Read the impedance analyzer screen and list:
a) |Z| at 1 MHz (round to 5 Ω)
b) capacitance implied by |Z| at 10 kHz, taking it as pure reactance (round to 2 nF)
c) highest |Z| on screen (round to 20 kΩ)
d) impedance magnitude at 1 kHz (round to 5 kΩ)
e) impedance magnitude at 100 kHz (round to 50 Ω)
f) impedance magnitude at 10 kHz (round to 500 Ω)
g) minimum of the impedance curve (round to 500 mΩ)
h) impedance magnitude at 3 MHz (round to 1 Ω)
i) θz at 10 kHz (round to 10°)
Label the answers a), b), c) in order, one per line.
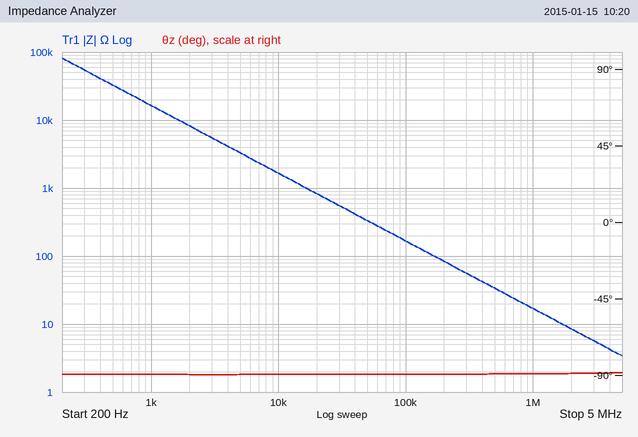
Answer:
a) 15 Ω
b) 10 nF
c) 80 kΩ
d) 15 kΩ
e) 150 Ω
f) 1.5 kΩ
g) 3.5 Ω
h) 6 Ω
i) -90°
